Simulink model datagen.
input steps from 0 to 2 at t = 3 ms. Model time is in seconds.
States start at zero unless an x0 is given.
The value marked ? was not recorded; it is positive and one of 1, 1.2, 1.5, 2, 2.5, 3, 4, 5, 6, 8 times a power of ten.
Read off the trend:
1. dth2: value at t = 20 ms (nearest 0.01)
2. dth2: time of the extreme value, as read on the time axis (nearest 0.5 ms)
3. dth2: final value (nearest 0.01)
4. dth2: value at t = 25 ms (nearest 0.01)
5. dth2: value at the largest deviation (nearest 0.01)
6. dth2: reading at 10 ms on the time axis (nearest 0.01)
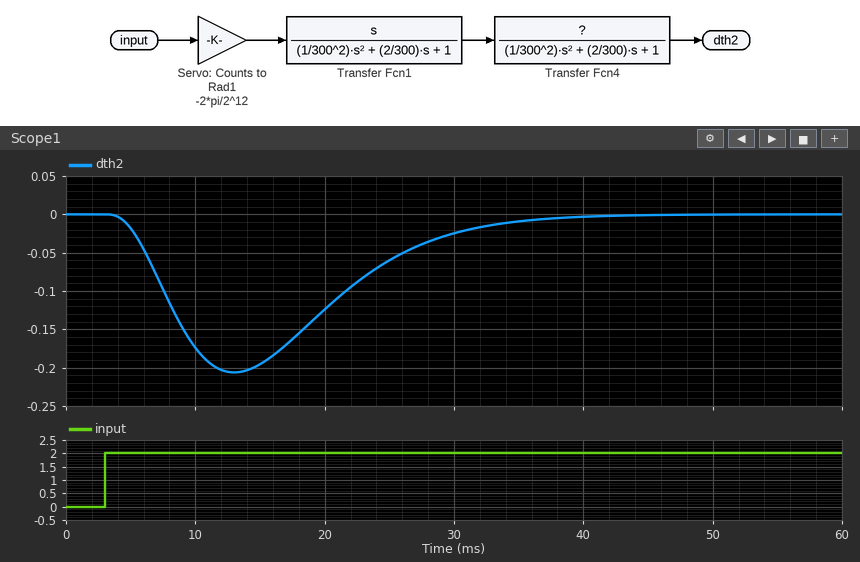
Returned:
-0.12
13.0 ms
0.00
-0.06
-0.21
-0.17
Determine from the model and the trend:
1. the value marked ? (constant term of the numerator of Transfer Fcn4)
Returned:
1
